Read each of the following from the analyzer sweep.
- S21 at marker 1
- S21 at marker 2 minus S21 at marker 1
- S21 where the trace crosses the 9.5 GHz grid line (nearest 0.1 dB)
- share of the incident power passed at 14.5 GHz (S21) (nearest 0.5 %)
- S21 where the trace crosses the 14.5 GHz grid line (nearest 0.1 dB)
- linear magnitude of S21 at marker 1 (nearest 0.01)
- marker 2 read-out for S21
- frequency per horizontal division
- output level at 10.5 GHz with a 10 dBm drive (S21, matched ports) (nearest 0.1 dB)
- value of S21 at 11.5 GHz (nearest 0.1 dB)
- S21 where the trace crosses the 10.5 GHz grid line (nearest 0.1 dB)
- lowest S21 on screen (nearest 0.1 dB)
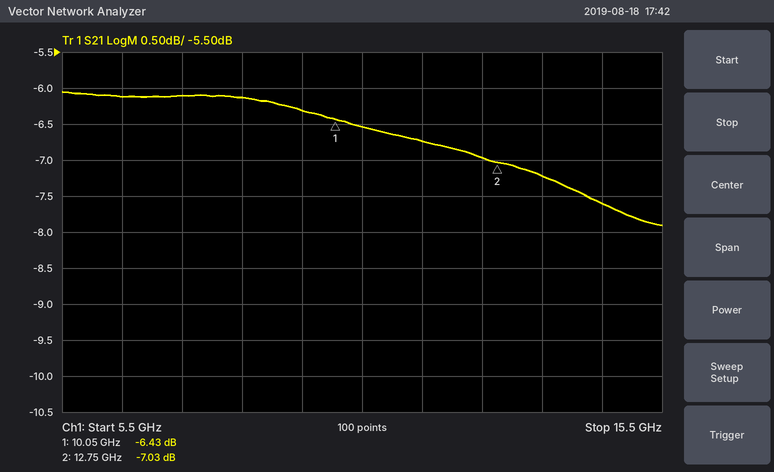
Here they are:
-6.43 dB
-0.60 dB
-6.3 dB
17.5 %
-7.6 dB
0.48
-7.03 dB
1 GHz
3.5 dBm
-6.7 dB
-6.5 dB
-7.9 dB
